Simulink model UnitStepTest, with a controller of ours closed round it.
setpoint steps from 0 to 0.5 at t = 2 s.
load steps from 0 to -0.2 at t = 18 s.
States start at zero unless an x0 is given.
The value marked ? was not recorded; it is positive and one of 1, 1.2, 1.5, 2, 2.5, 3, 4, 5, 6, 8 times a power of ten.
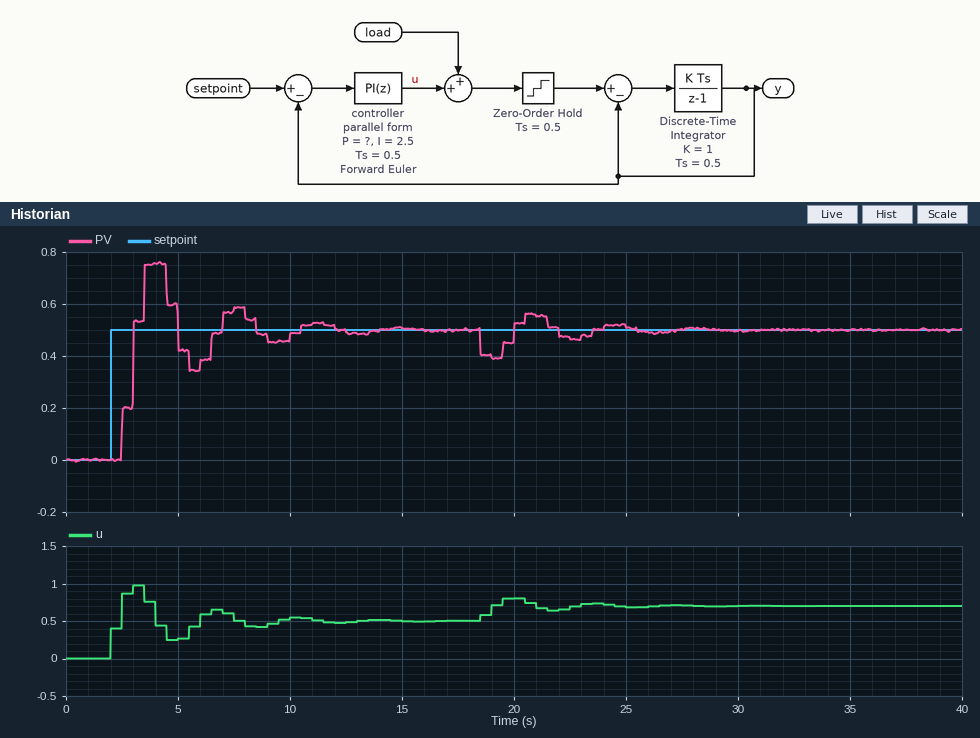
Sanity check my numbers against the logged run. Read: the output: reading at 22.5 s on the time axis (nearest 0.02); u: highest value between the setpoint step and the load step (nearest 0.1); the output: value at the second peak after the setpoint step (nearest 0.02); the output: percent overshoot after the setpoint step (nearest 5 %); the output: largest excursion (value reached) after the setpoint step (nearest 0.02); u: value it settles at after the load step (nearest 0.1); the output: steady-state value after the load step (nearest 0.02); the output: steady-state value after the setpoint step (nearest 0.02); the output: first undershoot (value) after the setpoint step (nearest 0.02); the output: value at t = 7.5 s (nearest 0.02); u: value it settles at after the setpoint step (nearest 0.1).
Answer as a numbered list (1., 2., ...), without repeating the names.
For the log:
1. 0.46
2. 1.0
3. 0.58
4. 50 %
5. 0.76
6. 0.7
7. 0.50
8. 0.50
9. 0.34
10. 0.58
11. 0.5
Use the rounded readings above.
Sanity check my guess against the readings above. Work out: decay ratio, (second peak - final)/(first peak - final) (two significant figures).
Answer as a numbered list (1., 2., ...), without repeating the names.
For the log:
1. 0.31
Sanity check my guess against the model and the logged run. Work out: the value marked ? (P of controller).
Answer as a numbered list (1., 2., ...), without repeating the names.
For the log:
1. 0.8
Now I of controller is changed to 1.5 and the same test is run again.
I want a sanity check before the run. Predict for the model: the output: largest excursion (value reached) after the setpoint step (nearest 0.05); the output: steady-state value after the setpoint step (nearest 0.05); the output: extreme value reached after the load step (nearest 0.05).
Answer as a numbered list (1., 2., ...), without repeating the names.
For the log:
1. 0.60
2. 0.50
3. 0.40
